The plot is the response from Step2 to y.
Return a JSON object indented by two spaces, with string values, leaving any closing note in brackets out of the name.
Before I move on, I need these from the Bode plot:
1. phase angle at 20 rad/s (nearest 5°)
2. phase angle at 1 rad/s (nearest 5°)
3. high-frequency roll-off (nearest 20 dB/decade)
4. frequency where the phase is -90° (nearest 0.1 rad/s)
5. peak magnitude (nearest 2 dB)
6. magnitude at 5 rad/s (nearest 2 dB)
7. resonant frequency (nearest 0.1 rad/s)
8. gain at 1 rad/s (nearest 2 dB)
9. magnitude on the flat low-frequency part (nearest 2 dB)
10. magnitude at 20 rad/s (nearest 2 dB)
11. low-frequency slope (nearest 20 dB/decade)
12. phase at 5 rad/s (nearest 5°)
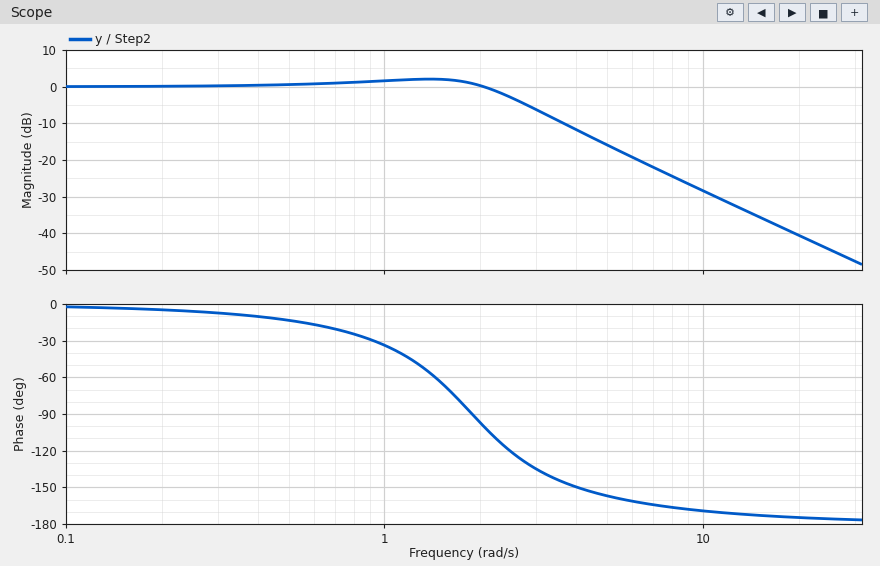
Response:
{
  "phase angle at 20 rad/s": "-175°",
  "phase angle at 1 rad/s": "-35°",
  "high-frequency roll-off": "-40 dB/decade",
  "frequency where the phase is -90°": "1.9 rad/s",
  "peak magnitude": "2 dB",
  "magnitude at 5 rad/s": "-16 dB",
  "resonant frequency": "1.3 rad/s",
  "gain at 1 rad/s": "2 dB",
  "magnitude on the flat low-frequency part": "0 dB",
  "magnitude at 20 rad/s": "-40 dB",
  "low-frequency slope": "0 dB/decade",
  "phase at 5 rad/s": "-155°"
}
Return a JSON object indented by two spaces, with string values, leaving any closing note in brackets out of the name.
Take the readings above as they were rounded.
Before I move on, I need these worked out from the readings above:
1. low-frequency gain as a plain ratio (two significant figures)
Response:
{
  "low-frequency gain as a plain ratio": "1.0"
}
